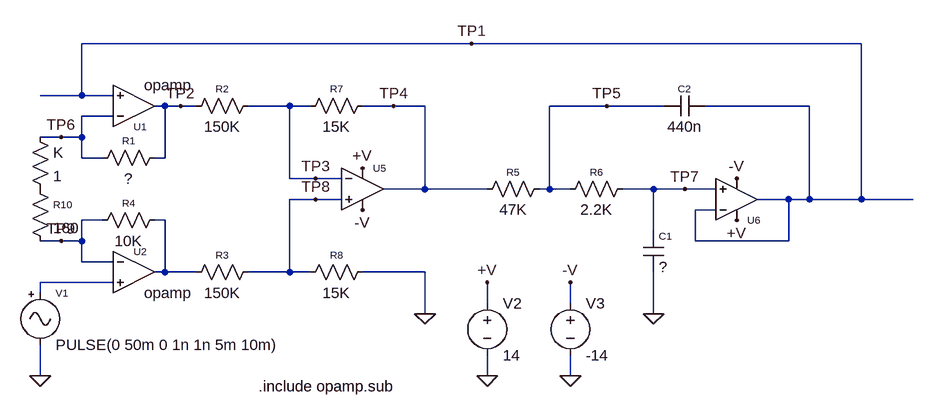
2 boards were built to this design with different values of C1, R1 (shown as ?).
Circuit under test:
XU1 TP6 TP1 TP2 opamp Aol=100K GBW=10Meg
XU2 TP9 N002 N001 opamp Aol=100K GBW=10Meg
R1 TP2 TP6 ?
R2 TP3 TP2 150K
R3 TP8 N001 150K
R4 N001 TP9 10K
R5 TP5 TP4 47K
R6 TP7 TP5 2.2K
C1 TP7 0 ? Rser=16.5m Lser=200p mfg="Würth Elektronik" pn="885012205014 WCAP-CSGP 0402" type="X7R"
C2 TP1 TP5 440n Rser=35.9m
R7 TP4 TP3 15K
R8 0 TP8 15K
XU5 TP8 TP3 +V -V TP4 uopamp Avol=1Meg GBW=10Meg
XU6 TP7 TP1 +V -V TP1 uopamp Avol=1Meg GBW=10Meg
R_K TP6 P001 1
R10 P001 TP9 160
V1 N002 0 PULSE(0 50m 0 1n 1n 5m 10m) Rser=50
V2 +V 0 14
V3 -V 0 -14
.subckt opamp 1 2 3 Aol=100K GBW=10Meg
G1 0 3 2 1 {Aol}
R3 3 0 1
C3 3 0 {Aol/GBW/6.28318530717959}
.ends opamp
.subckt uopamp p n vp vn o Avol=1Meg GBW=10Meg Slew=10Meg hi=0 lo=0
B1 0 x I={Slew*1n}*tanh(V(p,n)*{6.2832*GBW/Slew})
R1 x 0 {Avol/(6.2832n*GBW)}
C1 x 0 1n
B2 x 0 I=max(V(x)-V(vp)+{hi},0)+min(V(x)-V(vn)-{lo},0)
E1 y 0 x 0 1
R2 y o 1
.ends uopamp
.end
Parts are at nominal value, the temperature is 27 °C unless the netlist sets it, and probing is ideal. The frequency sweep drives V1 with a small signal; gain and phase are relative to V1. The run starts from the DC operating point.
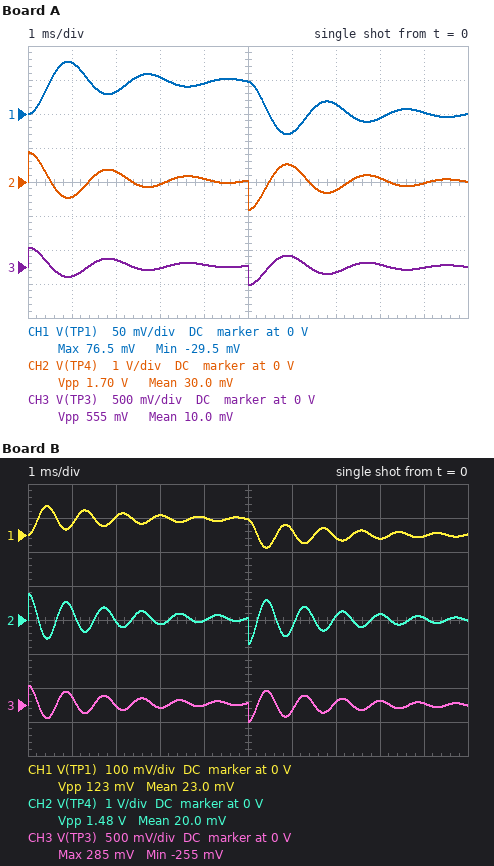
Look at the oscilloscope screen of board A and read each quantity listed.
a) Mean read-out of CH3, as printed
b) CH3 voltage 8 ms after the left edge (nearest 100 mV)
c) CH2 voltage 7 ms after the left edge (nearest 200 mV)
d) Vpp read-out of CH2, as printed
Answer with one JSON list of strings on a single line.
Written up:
["10.0 mV", "0 V", "-200 mV", "1.70 V"]
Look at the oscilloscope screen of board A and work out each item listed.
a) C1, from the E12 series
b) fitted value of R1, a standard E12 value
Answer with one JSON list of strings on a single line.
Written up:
["33 nF", "18 kΩ"]
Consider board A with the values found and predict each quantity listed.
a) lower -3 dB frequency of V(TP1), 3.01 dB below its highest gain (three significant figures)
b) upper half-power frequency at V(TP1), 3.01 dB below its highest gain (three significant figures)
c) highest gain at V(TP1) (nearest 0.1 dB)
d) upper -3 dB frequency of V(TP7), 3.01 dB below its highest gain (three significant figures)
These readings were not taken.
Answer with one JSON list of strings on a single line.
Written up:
["453 Hz", "624 Hz", "10.1 dB", "624 Hz"]
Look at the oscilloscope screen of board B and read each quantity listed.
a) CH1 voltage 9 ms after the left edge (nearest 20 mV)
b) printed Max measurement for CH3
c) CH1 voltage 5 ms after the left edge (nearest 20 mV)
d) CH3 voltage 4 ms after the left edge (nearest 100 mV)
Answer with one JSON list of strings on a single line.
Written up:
["0 V", "285 mV", "40 mV", "0 V"]
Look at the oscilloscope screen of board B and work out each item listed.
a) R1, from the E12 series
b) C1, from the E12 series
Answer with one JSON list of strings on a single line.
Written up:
["15 kΩ", "6.8 nF"]
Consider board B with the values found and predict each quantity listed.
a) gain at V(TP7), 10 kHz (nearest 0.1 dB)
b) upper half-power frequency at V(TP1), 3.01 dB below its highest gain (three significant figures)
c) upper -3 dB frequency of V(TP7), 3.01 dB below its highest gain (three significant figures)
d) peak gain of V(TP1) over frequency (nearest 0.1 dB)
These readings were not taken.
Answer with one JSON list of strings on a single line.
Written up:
["-37.9 dB", "1.23 kHz", "1.23 kHz", "17.2 dB"]
